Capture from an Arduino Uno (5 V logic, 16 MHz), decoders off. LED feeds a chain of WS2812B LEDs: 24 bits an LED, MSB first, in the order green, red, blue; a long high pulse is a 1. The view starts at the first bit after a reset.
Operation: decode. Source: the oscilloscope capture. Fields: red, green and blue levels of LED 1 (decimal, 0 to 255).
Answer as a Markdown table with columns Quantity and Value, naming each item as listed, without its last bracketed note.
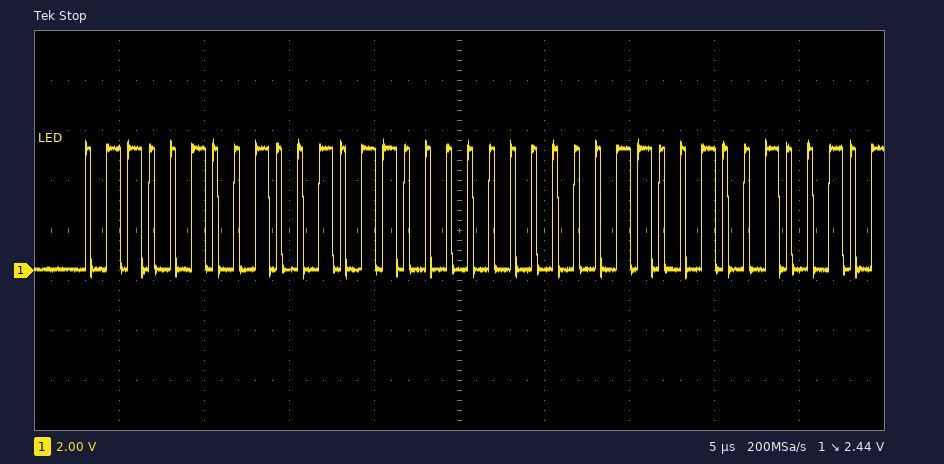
| Quantity | Value |
|---|---|
| red, green and blue levels of LED 1 | 150, 100, 0 |
